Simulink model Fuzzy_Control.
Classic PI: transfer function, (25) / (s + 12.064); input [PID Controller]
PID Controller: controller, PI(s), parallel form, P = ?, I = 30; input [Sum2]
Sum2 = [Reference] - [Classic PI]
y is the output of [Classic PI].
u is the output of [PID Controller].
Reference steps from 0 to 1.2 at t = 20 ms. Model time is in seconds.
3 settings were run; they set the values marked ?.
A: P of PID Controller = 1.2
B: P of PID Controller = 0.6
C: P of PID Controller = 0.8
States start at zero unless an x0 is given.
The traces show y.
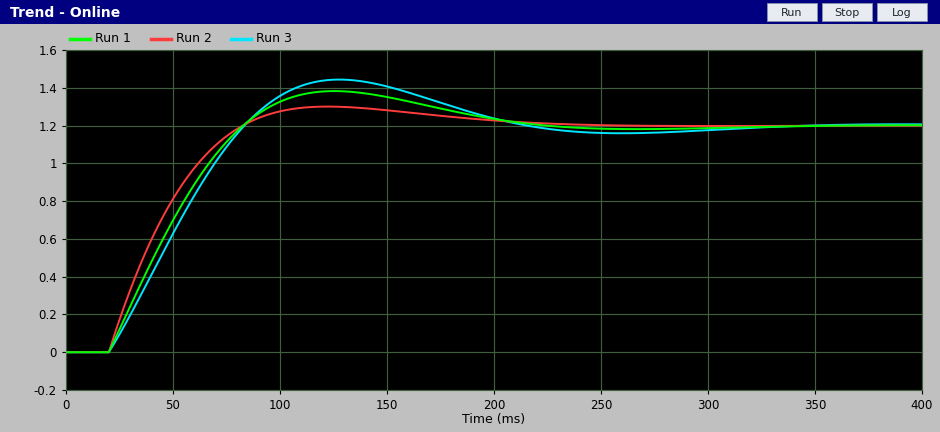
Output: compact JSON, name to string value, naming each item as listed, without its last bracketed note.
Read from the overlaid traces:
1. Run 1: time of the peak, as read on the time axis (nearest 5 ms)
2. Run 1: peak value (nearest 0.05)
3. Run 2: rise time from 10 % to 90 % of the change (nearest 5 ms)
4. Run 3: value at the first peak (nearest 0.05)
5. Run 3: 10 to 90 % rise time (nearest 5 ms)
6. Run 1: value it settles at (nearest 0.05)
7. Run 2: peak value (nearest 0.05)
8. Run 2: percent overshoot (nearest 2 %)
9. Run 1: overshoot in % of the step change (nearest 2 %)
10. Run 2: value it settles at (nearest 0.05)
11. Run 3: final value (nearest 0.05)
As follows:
{"Run 1: time of the peak, as read on the time axis": "125 ms", "Run 1: peak value": "1.40", "Run 2: rise time from 10 % to 90 % of the change": "45 ms", "Run 3: value at the first peak": "1.45", "Run 3: 10 to 90 % rise time": "50 ms", "Run 1: value it settles at": "1.20", "Run 2: peak value": "1.30", "Run 2: percent overshoot": "8 %", "Run 1: overshoot in % of the step change": "16 %", "Run 2: value it settles at": "1.20", "Run 3: final value": "1.20"}
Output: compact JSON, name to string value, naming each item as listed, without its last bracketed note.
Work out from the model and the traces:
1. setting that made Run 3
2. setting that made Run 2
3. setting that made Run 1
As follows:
{"setting that made Run 3": "B", "setting that made Run 2": "A", "setting that made Run 1": "C"}
